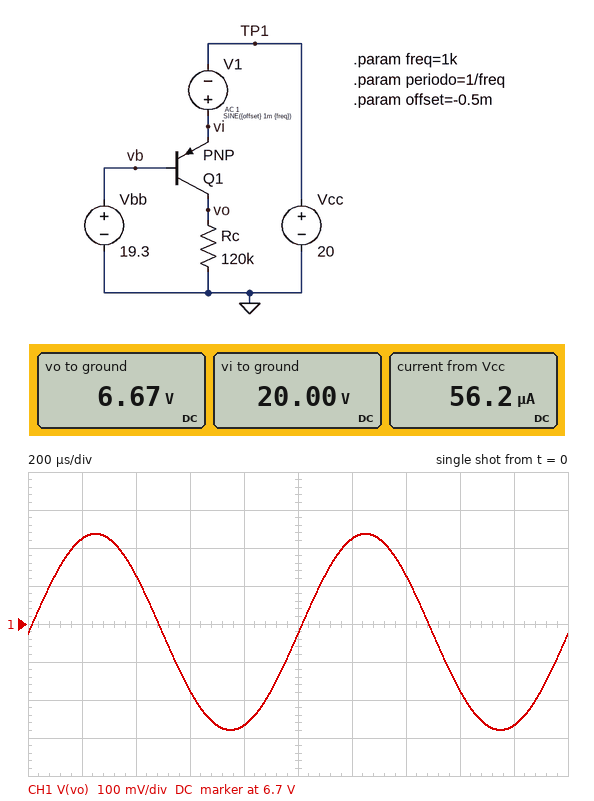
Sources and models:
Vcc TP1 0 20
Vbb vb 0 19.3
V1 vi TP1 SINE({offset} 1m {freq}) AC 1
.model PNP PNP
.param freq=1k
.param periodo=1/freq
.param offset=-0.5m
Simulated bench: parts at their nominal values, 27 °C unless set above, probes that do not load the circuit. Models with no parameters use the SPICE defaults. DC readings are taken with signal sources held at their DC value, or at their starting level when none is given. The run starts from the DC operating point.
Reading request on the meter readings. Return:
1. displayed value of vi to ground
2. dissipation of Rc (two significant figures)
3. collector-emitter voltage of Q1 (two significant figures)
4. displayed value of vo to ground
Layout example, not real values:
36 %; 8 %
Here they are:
20.00 V; 370 µW; -13 V; 6.67 V
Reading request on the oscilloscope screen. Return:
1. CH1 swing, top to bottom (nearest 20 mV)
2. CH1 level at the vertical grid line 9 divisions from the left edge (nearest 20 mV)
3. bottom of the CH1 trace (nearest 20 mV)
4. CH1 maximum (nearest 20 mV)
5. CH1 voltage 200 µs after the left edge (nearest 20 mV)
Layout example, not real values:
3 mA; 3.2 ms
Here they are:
520 mV; 6.44 V; 6.42 V; 6.94 V; 6.92 V
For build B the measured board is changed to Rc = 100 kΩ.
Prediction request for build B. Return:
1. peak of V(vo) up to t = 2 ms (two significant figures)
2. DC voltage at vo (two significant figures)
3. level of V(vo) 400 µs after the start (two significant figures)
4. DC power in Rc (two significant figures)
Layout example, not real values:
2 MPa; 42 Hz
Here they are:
5.8 V; 5.6 V; 5.7 V; 310 µW
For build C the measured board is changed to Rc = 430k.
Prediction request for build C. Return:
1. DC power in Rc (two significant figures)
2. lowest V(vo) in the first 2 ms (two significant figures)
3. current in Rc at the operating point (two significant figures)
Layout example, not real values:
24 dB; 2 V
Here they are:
920 µW; 20 V; 46 µA
